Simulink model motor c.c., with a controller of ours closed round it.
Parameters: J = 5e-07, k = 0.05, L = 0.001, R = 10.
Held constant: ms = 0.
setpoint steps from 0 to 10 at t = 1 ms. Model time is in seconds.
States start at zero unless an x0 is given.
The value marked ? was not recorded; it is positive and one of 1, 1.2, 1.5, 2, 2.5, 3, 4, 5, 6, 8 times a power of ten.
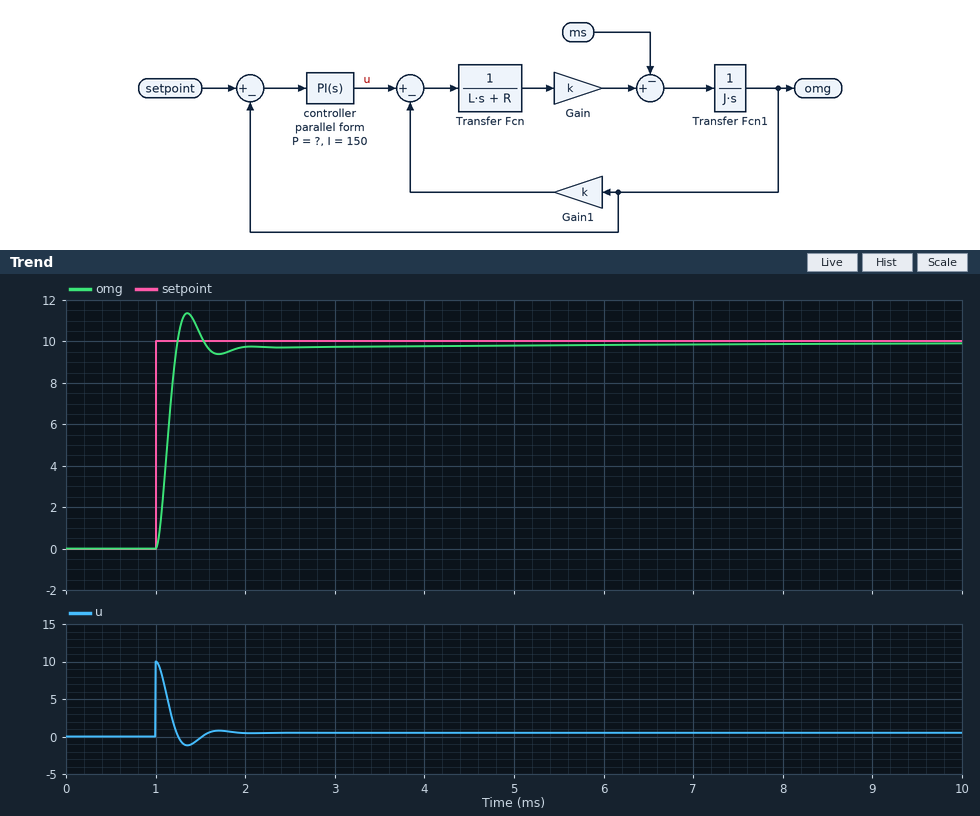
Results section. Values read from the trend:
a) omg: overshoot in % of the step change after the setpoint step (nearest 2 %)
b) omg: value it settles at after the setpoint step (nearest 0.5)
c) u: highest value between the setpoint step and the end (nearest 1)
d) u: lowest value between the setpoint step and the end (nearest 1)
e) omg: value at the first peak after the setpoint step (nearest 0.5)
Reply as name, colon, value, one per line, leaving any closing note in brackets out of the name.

omg: overshoot in % of the step change after the setpoint step: 14 %
omg: value it settles at after the setpoint step: 10.0
u: highest value between the setpoint step and the end: 10
u: lowest value between the setpoint step and the end: -1
omg: value at the first peak after the setpoint step: 11.5
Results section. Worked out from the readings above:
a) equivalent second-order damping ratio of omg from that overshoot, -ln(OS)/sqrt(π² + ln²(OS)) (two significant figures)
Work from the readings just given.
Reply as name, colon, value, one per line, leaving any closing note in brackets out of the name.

equivalent second-order damping ratio of omg from that overshoot, -ln(OS)/sqrt(π² + ln²(OS)): 0.53
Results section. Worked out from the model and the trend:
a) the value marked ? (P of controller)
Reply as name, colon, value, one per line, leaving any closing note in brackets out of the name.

the value marked ?: 1
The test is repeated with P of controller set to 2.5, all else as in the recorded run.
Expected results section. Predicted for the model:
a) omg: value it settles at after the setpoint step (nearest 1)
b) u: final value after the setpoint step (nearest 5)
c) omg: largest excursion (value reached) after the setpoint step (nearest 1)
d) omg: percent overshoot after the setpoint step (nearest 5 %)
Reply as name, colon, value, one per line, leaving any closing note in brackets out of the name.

omg: value it settles at after the setpoint step: 10
u: final value after the setpoint step: 0
omg: largest excursion (value reached) after the setpoint step: 13
omg: percent overshoot after the setpoint step: 35 %
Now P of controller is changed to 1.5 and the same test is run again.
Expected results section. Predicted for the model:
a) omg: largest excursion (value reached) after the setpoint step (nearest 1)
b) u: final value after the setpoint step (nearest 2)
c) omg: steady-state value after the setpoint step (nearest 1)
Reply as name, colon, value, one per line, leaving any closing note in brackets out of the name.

omg: largest excursion (value reached) after the setpoint step: 12
u: final value after the setpoint step: 0
omg: steady-state value after the setpoint step: 10
